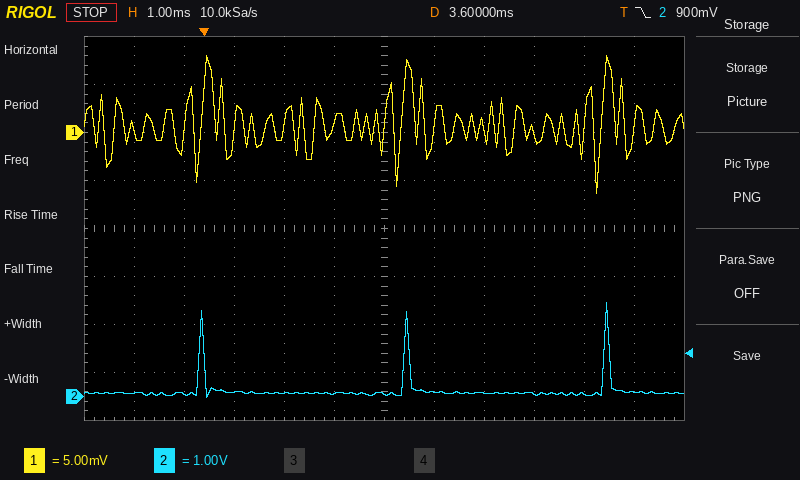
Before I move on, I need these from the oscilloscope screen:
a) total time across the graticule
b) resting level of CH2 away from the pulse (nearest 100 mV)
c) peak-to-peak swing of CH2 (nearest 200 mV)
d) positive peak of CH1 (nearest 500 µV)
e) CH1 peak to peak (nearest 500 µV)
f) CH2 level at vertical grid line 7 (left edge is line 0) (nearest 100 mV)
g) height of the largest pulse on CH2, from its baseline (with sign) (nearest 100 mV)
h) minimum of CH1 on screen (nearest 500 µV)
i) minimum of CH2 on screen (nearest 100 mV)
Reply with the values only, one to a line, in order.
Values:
12 ms
100 mV
2.0 V
8.0 mV
14.5 mV
100 mV
+1.9 V
-6.5 mV
0.0 V
